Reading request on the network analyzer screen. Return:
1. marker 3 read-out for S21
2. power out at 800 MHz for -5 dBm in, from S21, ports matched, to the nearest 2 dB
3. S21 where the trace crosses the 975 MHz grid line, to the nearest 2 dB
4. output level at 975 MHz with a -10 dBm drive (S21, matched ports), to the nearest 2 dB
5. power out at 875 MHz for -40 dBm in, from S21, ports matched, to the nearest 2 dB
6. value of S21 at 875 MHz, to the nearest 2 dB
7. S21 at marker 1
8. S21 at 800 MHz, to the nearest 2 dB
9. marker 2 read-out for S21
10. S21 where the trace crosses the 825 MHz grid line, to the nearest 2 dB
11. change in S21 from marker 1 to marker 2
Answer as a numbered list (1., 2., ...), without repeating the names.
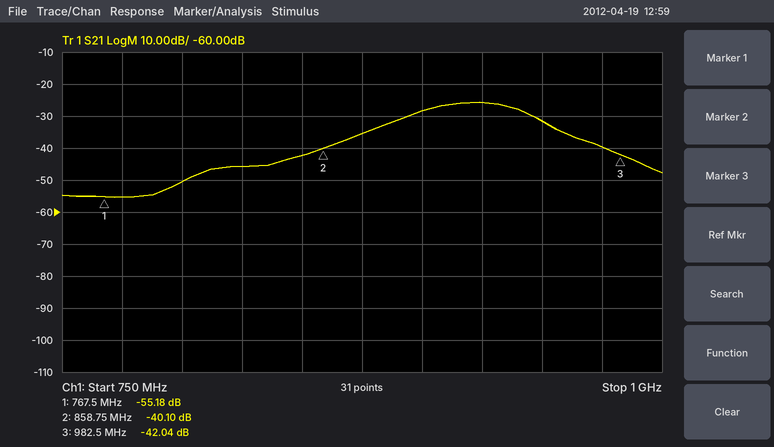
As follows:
1. -42.04 dB
2. -56 dBm
3. -40 dB
4. -50 dBm
5. -76 dBm
6. -36 dB
7. -55.18 dB
8. -50 dB
9. -40.10 dB
10. -46 dB
11. 15.08 dB
